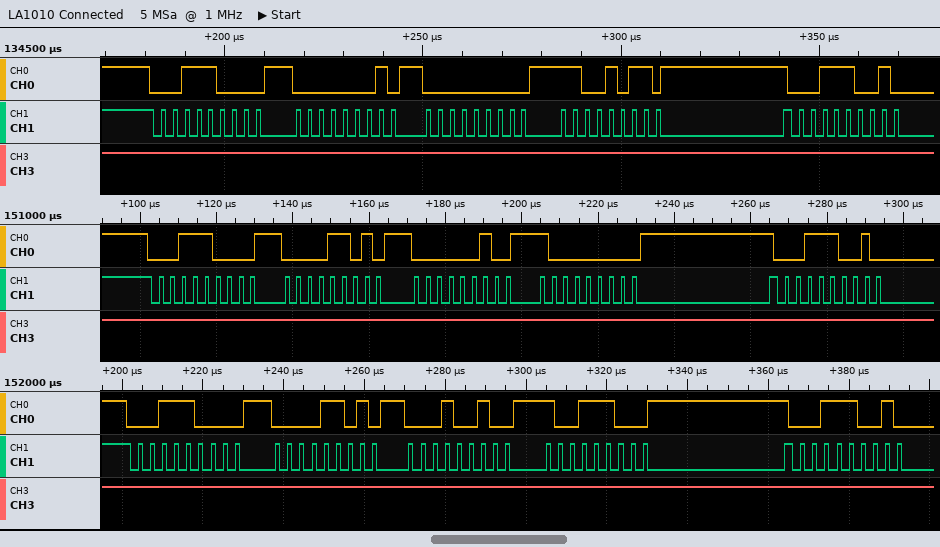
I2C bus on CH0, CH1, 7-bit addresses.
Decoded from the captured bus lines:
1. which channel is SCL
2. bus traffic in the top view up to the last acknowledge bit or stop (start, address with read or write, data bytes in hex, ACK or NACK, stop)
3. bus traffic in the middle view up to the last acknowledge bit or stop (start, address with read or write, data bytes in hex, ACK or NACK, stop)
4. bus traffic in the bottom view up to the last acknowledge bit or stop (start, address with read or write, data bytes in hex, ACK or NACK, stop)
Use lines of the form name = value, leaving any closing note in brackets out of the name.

which channel is SCL = CH1
bus traffic in the top view up to the last acknowledge bit or stop = start, address 1C write ACK, 01 ACK, 00 ACK, CB ACK, repeated start, address 1C read ACK
bus traffic in the middle view up to the last acknowledge bit or stop = start, address 1C write ACK, 0D ACK, 02 ACK, 80 ACK, repeated start, address 1C read ACK
bus traffic in the bottom view up to the last acknowledge bit or stop = start, address 1C write ACK, 0D ACK, 12 ACK, 9C ACK, repeated start, address 1C read ACK
